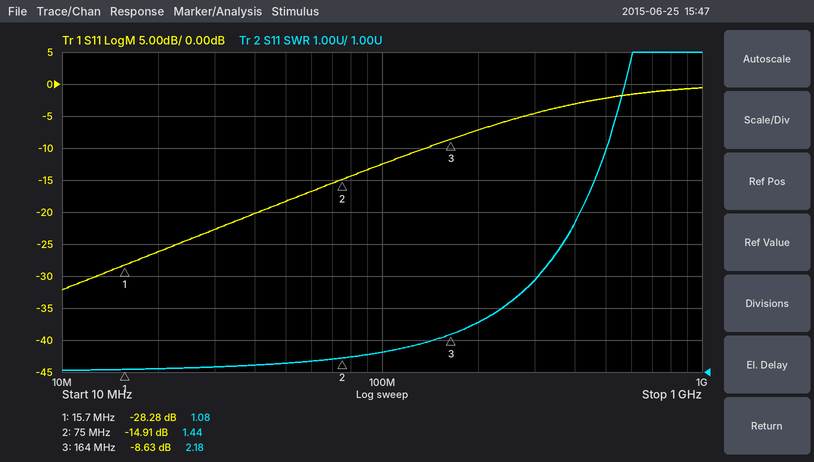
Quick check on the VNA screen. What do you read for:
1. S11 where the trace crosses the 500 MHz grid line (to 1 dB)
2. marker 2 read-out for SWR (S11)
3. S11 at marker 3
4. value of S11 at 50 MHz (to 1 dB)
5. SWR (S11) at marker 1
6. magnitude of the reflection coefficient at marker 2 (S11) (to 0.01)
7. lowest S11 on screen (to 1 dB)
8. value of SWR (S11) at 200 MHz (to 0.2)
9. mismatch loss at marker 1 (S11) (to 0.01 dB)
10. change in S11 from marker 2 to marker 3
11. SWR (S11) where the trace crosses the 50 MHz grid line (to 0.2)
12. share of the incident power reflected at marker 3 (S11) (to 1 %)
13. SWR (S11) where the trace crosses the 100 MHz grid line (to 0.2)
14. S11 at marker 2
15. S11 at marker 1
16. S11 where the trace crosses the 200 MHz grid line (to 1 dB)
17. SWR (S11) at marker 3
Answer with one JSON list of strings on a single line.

["-2 dB", "1.44", "-8.63 dB", "-18 dB", "1.08", "0.18", "-32 dB", "2.6", "0.01 dB", "6.28 dB", "1.2", "14 %", "1.6", "-14.91 dB", "-28.28 dB", "-7 dB", "2.18"]
